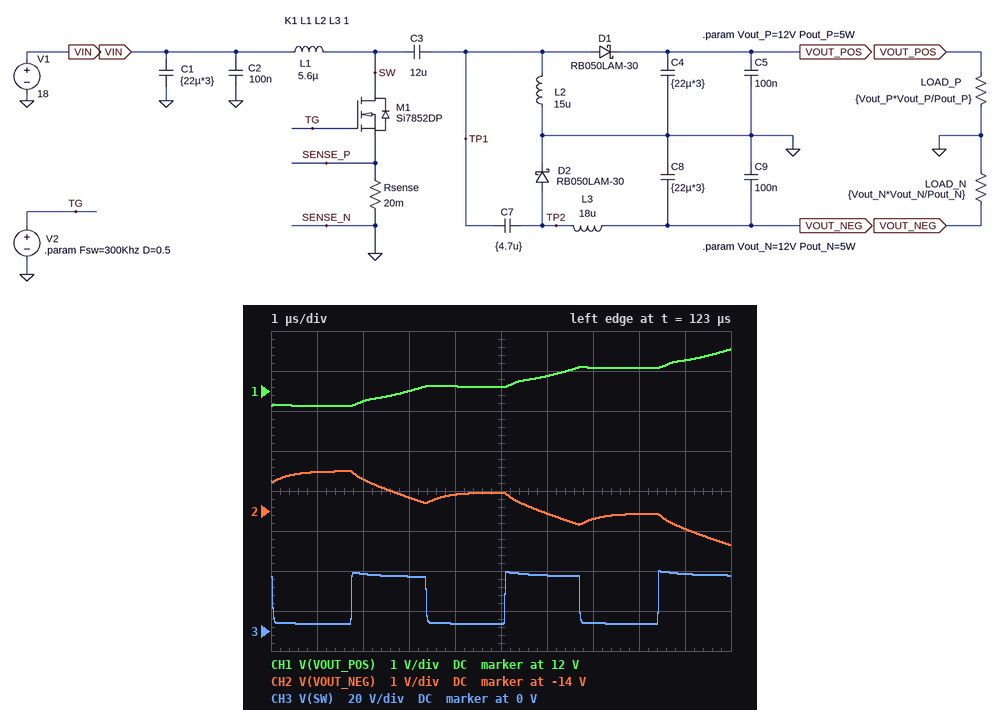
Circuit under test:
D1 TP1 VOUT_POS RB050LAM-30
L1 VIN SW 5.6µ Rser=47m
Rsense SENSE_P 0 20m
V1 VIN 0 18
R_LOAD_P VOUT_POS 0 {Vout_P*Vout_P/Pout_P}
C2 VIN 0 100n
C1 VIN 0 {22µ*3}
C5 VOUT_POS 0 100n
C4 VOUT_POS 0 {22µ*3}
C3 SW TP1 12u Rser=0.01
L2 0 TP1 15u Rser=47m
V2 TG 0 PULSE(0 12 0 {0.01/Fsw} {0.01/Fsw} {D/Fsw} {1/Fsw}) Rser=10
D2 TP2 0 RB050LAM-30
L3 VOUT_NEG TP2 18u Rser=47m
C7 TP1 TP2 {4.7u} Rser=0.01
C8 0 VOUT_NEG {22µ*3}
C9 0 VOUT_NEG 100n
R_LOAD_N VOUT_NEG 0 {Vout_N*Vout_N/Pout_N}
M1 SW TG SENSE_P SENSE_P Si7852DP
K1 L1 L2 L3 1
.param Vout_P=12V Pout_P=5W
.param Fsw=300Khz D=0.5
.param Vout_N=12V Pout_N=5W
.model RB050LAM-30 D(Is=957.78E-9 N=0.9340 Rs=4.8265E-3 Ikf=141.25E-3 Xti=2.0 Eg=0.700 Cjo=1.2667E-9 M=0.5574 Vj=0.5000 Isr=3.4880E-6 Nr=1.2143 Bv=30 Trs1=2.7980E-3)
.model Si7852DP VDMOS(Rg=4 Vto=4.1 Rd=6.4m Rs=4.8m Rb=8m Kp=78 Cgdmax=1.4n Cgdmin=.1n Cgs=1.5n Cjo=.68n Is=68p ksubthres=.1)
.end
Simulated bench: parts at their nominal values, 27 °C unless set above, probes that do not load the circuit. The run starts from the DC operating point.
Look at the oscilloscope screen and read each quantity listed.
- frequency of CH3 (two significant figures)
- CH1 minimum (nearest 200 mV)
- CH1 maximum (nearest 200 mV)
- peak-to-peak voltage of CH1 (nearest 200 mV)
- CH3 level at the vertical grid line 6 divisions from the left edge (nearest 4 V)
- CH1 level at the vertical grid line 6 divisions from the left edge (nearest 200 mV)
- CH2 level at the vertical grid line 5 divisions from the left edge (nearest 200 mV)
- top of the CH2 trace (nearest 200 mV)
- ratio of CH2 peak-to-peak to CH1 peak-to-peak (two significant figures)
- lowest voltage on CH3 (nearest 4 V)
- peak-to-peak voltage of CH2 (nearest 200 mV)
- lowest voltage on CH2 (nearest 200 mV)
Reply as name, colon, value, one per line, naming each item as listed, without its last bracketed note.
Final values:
frequency of CH3: 300 kHz
CH1 minimum: 11.6 V
CH1 maximum: 13.0 V
peak-to-peak voltage of CH1: 1.4 V
CH3 level at the vertical grid line 6 divisions from the left edge: 28 V
CH1 level at the vertical grid line 6 divisions from the left edge: 12.4 V
CH2 level at the vertical grid line 5 divisions from the left edge: -13.6 V
top of the CH2 trace: -13.0 V
ratio of CH2 peak-to-peak to CH1 peak-to-peak: 1.3
lowest voltage on CH3: 4 V
peak-to-peak voltage of CH2: 1.8 V
lowest voltage on CH2: -14.8 V
